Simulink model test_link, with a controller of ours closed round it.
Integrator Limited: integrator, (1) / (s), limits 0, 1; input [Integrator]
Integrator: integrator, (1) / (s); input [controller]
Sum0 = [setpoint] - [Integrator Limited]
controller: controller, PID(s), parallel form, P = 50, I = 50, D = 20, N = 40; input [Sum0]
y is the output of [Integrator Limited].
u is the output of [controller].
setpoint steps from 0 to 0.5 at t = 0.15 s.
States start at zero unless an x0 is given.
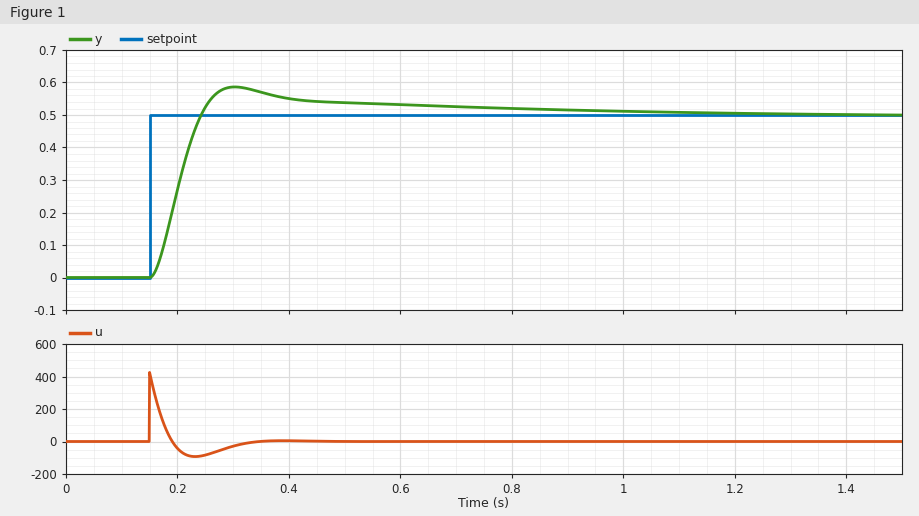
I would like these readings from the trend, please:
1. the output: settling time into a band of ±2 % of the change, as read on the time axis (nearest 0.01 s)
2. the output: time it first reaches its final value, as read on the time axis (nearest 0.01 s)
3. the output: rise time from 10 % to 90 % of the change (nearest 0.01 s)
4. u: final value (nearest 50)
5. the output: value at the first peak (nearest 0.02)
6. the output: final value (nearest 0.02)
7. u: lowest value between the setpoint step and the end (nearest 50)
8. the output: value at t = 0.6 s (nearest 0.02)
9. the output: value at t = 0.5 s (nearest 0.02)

1.04 s
0.24 s
0.06 s
0
0.58
0.50
-100
0.54
0.54
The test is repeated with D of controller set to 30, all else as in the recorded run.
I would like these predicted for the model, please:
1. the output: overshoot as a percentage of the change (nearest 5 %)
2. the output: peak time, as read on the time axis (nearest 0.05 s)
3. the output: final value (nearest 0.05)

20 %
0.25 s
0.50
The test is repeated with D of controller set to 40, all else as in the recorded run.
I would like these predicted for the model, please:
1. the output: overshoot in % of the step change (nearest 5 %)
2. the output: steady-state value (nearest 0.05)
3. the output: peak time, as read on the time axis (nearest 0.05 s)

20 %
0.50
0.25 s
